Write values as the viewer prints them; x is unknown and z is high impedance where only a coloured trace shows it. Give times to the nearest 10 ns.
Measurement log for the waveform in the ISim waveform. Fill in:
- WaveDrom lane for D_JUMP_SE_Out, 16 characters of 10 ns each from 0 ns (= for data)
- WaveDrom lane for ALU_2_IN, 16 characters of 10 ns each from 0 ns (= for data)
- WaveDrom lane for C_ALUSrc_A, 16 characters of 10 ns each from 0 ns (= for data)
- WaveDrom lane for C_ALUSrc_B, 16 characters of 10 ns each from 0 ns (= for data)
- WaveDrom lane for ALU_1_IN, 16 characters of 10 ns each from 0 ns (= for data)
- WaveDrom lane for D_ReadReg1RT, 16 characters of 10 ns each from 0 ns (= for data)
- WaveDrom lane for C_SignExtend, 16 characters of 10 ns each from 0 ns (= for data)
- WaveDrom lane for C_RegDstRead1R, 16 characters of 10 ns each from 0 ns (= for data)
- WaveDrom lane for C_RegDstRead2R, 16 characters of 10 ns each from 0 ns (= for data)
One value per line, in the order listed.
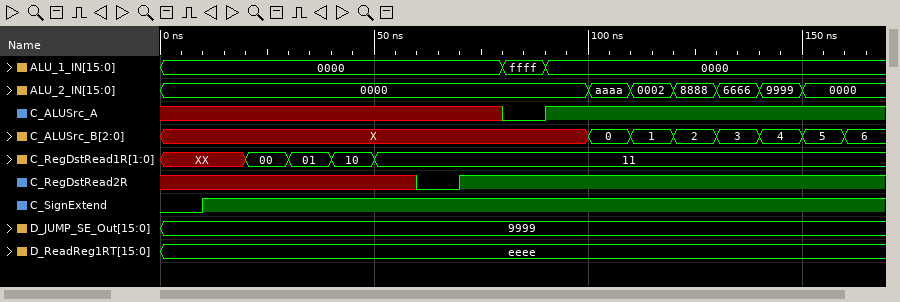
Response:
{name: 'D_JUMP_SE_Out', wave: '=...............', data: '9999'}
{name: 'ALU_2_IN', wave: '=.........======', data: '0000 aaaa 0002 8888 6666 9999 0000'}
{name: 'C_ALUSrc_A', wave: 'x.......01......'}
{name: 'C_ALUSrc_B', wave: 'x.........======', data: '0 1 2 3 4 5'}
{name: 'ALU_1_IN', wave: '=.......==......', data: '0000 ffff 0000'}
{name: 'D_ReadReg1RT', wave: '=...............', data: 'eeee'}
{name: 'C_SignExtend', wave: '01..............'}
{name: 'C_RegDstRead1R', wave: 'x.====..........', data: '00 01 10 11'}
{name: 'C_RegDstRead2R', wave: 'x.....01........'}
